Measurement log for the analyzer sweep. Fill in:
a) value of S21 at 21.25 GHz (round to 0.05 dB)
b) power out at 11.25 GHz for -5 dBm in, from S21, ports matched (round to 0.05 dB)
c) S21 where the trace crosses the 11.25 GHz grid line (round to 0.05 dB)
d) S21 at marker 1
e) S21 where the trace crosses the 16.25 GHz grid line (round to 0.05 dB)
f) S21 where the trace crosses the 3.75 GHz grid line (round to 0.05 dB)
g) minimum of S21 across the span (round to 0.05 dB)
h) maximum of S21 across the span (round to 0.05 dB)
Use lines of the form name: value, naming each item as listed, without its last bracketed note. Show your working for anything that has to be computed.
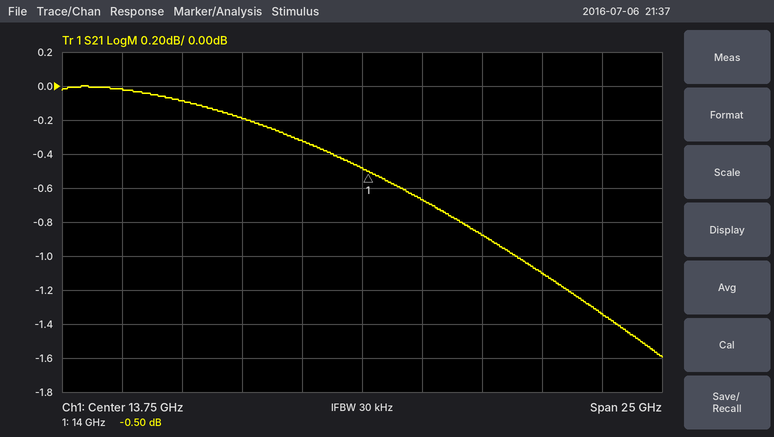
value of S21 at 21.25 GHz: -1.10 dB
power out at 11.25 GHz for -5 dBm in, from S21, ports matched: -5 dBm + (-0.30 dB) = -5.30 dBm
S21 where the trace crosses the 11.25 GHz grid line: -0.30 dB
S21 at marker 1: -0.50 dB
S21 where the trace crosses the 16.25 GHz grid line: -0.65 dB
S21 where the trace crosses the 3.75 GHz grid line: 0.00 dB
minimum of S21 across the span: -1.60 dB
maximum of S21 across the span: 0.00 dB
